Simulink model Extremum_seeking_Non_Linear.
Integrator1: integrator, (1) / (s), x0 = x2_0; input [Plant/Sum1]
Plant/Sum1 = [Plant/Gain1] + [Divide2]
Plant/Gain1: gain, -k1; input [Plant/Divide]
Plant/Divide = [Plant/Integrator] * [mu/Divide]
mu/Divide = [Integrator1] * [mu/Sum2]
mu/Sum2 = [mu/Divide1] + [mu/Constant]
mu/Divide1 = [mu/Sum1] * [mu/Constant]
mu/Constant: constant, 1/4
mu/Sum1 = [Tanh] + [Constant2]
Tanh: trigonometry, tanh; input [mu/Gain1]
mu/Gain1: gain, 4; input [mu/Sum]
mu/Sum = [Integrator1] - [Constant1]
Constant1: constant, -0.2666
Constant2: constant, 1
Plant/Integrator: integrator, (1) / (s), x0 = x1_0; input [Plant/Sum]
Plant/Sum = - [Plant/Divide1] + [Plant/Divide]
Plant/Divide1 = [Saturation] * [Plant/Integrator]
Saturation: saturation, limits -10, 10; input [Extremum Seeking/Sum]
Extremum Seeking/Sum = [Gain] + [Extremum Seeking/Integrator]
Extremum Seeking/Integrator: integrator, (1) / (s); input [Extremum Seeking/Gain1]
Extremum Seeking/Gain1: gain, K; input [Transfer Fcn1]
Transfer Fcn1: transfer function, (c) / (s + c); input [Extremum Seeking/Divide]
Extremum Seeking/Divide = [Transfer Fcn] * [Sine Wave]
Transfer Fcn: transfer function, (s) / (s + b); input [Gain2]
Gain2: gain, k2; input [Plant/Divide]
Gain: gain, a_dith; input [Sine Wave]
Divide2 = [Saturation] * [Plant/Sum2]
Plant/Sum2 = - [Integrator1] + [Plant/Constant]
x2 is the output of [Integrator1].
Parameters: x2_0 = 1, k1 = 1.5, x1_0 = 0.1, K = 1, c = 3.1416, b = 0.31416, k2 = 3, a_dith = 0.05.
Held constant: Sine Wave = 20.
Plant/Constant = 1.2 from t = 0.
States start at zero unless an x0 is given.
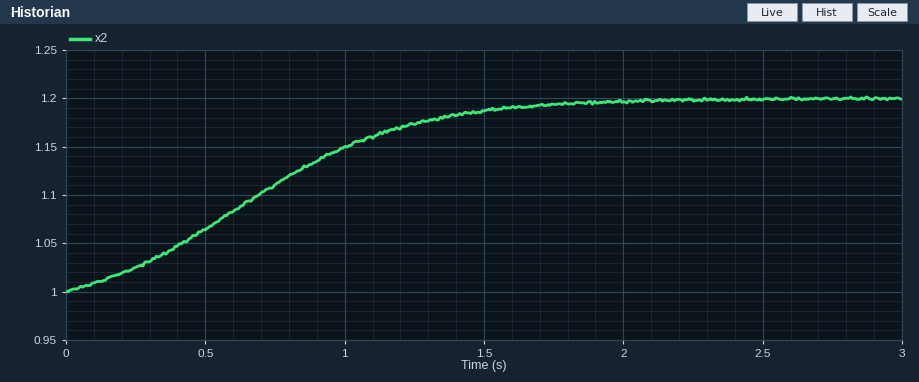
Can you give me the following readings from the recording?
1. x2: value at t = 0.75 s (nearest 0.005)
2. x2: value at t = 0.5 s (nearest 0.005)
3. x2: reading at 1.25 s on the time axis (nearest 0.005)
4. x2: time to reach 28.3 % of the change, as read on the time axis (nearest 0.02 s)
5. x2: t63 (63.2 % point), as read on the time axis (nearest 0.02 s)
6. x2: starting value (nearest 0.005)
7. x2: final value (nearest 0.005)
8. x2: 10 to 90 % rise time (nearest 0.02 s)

1.110
1.065
1.175
0.46 s
0.84 s
1.000
1.200
1.14 s
